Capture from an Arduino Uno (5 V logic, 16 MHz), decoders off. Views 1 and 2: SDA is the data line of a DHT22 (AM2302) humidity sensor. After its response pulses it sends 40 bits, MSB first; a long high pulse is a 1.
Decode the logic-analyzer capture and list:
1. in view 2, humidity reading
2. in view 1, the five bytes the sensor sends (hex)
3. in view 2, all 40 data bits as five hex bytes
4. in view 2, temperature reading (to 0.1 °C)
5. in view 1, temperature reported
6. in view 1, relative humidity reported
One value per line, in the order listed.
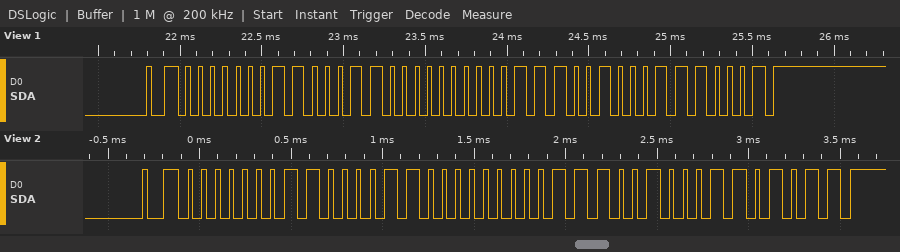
39.0 %
01 8C 00 E4 71
01 86 00 E4 6B
22.8 °C
22.8 °C
39.6 %
